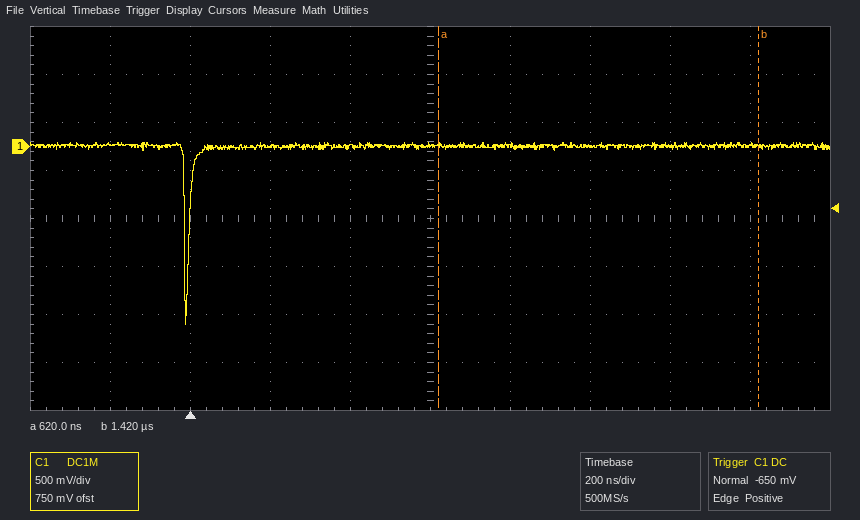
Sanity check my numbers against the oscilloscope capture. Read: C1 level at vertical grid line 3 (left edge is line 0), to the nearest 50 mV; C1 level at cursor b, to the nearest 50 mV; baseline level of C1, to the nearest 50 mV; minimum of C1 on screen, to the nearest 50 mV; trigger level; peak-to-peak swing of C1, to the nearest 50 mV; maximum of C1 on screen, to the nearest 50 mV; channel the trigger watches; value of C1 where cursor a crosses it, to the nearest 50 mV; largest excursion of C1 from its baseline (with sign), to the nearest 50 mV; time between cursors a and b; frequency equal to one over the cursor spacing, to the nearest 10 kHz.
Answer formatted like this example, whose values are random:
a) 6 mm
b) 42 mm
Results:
a) 0 mV
b) 0 mV
c) 0 mV
d) -1.85 V
e) -650 mV
f) 1.90 V
g) 50 mV
h) C1
i) 0 mV
j) -1.85 V
k) 800 ns
l) 1.25 MHz
